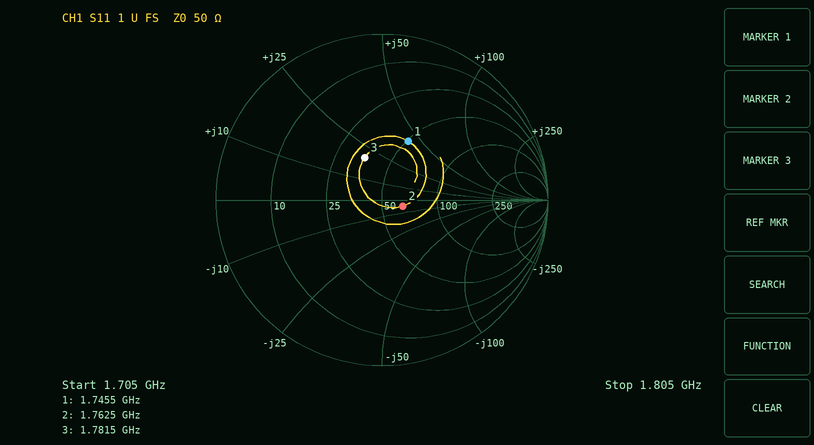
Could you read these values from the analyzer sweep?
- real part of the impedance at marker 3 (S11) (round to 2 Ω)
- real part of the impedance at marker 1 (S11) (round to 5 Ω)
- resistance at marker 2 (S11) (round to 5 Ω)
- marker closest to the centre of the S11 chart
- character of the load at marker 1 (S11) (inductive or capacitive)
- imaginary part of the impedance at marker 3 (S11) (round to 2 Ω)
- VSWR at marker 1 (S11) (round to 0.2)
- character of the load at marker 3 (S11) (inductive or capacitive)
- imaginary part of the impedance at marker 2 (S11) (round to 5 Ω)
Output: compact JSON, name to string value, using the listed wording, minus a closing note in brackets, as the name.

{"real part of the impedance at marker 3 (S11)": "36 Ω", "real part of the impedance at marker 1 (S11)": "50 Ω", "resistance at marker 2 (S11)": "65 Ω", "marker closest to the centre of the S11 chart": "marker 2", "character of the load at marker 1 (S11)": "inductive", "imaginary part of the impedance at marker 3 (S11)": "+20 Ω", "VSWR at marker 1 (S11)": "2.2", "character of the load at marker 3 (S11)": "inductive", "imaginary part of the impedance at marker 2 (S11)": "-5 Ω"}
